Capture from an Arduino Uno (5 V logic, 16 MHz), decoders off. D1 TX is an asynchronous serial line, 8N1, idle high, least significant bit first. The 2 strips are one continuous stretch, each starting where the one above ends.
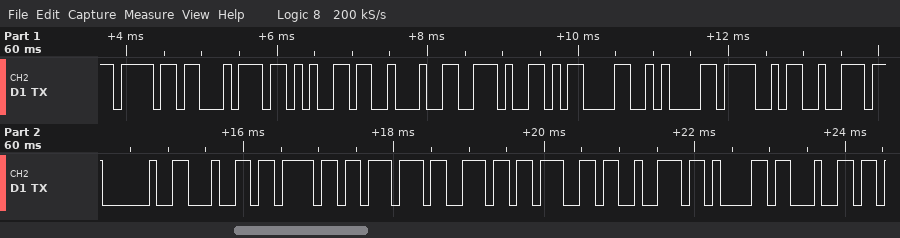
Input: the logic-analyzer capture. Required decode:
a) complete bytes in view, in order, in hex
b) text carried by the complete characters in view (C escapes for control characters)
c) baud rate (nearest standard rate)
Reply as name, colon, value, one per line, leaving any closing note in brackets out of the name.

complete bytes in view, in order, in hex: 0x6F 0x74 0x65 0x22 0x2E 0x0D 0x0A 0x4F 0x72 0x20 0x64 0x6F 0x77 0x6E 0x67 0x72 0x61 0x64
text carried by the complete characters in view: "ote\".\r\nOr downgrad"
baud rate: 9600 baud
